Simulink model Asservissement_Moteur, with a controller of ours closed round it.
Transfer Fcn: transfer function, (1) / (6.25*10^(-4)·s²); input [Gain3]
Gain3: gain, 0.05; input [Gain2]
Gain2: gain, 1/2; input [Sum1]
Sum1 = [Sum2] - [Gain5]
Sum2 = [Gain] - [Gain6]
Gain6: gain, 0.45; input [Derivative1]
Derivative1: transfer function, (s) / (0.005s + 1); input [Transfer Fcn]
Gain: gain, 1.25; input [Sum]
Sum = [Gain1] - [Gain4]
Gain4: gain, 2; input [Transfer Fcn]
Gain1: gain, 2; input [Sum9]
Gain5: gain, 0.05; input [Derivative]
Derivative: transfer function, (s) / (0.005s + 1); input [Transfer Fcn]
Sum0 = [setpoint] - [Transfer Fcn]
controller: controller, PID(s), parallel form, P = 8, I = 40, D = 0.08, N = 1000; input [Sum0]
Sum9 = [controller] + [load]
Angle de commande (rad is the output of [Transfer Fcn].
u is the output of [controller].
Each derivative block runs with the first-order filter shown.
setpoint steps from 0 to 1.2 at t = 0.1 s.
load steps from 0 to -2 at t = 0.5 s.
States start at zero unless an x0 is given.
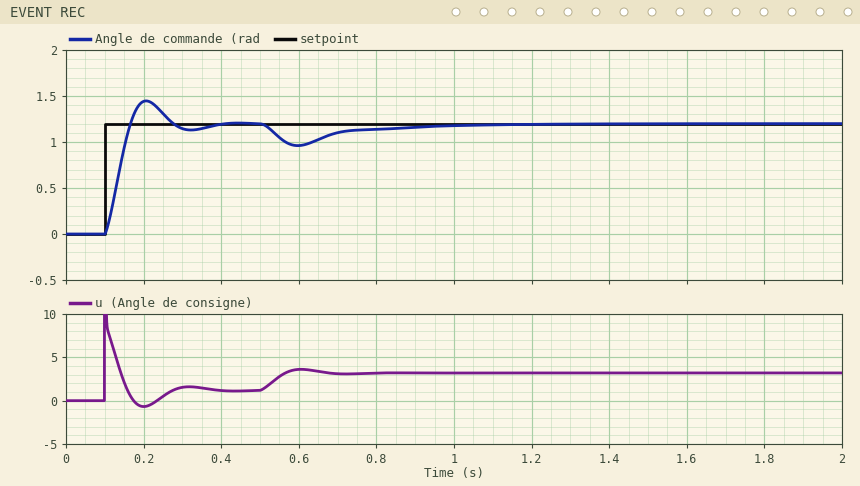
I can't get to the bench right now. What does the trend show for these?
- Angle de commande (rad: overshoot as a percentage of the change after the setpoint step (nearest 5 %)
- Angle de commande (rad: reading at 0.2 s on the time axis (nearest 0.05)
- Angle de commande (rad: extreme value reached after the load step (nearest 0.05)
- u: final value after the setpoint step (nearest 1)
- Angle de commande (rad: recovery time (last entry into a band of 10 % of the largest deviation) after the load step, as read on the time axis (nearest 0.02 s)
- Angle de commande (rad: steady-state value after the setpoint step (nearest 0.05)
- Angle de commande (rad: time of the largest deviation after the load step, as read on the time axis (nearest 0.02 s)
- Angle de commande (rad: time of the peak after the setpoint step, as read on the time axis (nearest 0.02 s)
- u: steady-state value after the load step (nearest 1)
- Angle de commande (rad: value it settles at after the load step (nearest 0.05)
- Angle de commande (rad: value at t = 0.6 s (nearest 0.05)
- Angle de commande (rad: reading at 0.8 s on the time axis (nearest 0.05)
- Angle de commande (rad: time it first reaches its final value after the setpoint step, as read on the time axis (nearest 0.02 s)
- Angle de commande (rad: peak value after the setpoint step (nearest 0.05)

20 %
1.45
0.95
1
0.98 s
1.20
0.60 s
0.20 s
3
1.20
0.95
1.15
0.16 s
1.45
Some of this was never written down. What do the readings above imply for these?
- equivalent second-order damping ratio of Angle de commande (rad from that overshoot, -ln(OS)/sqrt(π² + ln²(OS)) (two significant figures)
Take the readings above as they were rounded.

0.46
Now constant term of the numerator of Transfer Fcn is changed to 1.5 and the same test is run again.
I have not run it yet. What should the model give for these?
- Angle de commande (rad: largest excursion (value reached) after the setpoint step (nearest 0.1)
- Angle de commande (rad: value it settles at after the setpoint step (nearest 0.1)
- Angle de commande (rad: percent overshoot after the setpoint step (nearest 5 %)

1.3
1.2
10 %
